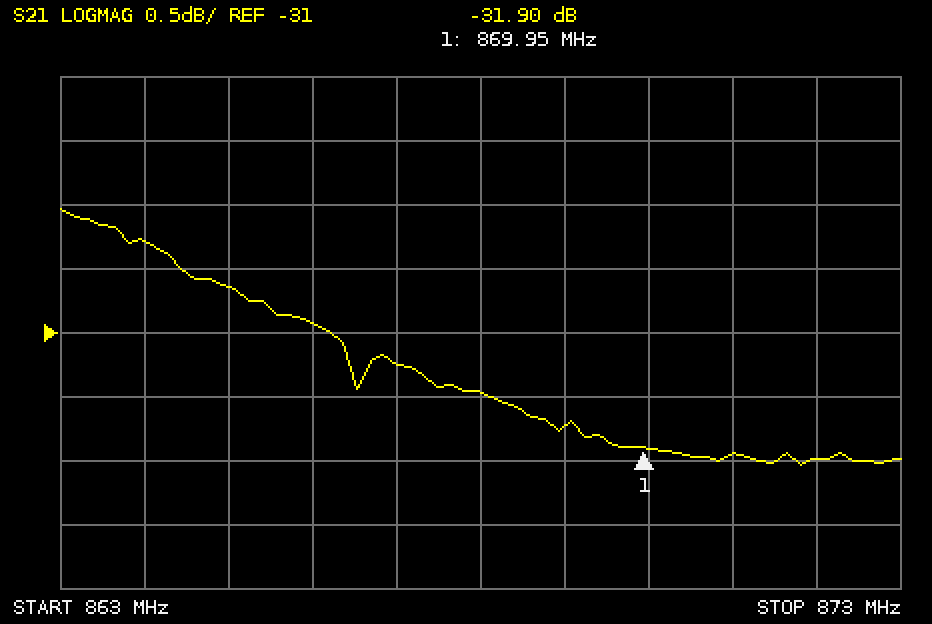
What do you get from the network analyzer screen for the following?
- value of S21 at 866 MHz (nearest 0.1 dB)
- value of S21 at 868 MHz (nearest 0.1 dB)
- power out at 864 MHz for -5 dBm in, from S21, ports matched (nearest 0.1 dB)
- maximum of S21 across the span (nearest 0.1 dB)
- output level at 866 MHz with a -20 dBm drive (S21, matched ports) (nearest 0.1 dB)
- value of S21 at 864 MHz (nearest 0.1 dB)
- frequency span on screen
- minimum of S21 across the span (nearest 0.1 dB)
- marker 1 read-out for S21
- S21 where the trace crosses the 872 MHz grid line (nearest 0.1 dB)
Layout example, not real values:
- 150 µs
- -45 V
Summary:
- -30.9 dB
- -31.5 dB
- -35.3 dBm
- -30.0 dB
- -50.9 dBm
- -30.3 dB
- 10 MHz
- -32.0 dB
- -31.90 dB
- -32.0 dB
